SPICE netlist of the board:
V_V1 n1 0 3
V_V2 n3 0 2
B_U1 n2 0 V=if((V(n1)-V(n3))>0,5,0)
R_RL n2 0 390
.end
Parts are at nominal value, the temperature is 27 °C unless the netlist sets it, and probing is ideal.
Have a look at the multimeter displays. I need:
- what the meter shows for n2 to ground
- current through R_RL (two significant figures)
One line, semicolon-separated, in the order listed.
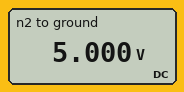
5.000 V; 13 mA
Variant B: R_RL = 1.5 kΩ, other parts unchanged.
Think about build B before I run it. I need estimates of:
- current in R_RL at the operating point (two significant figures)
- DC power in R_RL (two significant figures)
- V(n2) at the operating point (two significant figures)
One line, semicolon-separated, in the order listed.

3.3 mA; 17 mW; 5.0 V
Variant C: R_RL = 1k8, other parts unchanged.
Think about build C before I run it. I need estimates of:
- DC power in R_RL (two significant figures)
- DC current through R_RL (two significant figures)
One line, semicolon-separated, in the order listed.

14 mW; 2.8 mA
